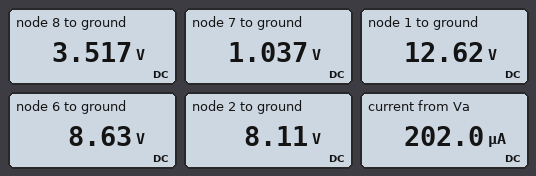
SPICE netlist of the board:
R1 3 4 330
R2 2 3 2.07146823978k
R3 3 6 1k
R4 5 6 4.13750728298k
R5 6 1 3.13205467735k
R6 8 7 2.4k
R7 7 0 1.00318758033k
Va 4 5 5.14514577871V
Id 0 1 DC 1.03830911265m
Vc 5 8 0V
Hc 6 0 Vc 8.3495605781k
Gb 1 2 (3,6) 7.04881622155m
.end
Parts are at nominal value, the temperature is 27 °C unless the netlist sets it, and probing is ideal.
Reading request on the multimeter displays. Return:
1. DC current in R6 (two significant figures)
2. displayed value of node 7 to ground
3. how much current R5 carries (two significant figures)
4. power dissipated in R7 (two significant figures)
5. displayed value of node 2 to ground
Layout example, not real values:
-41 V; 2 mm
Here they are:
1.0 mA; 1.037 V; 1.3 mA; 1.1 mW; 8.11 V
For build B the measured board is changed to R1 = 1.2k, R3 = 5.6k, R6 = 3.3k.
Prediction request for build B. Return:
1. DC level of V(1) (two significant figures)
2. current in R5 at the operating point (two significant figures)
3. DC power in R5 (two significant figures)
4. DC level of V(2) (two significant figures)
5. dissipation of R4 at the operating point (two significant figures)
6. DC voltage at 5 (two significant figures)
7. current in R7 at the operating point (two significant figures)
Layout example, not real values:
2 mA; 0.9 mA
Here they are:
14 V; 1.0 mA; 3.2 mW; 11 V; 6.5 mW; 5.5 V; 1.3 mA
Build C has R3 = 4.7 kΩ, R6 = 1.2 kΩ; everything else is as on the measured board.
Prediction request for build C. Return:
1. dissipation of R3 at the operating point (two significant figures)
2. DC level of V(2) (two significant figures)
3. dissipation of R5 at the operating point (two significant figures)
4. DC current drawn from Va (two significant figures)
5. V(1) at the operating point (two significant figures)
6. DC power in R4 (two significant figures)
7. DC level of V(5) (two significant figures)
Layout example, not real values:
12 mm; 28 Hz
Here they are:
730 nW; 6.0 V; 6.6 mW; 400 µA; 11 V; 6.2 mW; 1.8 V
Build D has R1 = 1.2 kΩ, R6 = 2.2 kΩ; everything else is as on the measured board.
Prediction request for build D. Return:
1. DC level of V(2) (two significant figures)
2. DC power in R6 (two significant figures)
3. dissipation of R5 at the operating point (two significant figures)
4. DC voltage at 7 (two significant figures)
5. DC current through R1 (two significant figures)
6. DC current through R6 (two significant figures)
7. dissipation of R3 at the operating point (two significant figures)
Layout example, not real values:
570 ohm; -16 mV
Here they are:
7.4 V; 2.0 mW; 5.4 mW; 960 mV; 230 µA; 950 µA; 1.5 µW
